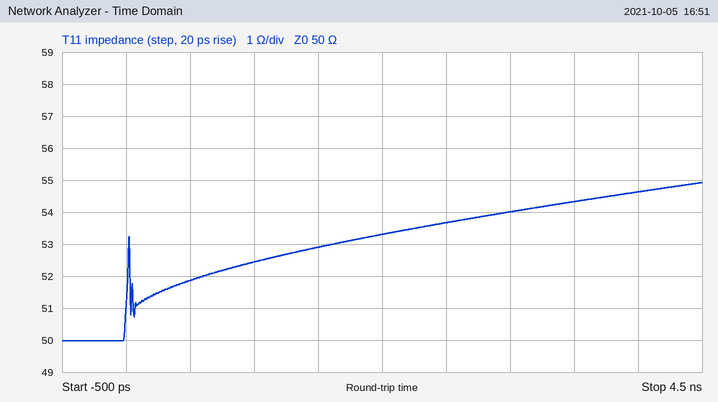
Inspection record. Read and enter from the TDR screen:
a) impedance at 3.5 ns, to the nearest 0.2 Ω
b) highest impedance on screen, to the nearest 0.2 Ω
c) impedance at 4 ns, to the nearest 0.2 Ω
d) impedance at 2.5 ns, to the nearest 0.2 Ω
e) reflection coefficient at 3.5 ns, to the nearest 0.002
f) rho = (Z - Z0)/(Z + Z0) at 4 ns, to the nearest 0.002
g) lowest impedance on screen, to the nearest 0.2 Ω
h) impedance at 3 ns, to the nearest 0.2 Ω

54.4 Ω
55.0 Ω
54.6 Ω
53.6 Ω
+0.042
+0.044
50.0 Ω
54.0 Ω
